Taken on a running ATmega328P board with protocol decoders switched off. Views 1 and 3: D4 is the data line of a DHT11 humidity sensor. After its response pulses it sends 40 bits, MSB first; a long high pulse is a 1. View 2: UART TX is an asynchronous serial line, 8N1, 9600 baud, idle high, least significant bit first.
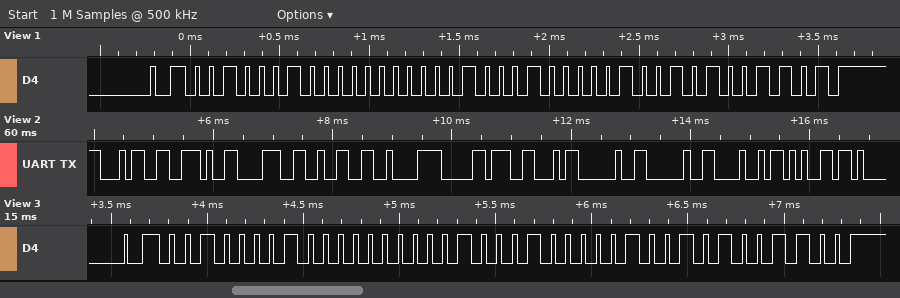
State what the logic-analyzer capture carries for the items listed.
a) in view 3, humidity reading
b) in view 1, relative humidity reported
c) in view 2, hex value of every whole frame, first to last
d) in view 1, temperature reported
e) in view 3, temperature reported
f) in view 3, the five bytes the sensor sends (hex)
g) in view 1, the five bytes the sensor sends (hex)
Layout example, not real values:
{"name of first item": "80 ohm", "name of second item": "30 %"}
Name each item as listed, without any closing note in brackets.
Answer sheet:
{"in view 3, humidity reading": "33 %", "in view 1, relative humidity reported": "34 %", "in view 2, hex value of every whole frame, first to last": "0x34 0x2E 0x38 0x32 0xC2 0xB0 0x46 0x20 0x20 0x48 0x65", "in view 1, temperature reported": "34.9 °C", "in view 3, temperature reported": "34.9 °C", "in view 3, the five bytes the sensor sends": "21 00 22 09 4C", "in view 1, the five bytes the sensor sends": "22 00 22 09 4D"}
